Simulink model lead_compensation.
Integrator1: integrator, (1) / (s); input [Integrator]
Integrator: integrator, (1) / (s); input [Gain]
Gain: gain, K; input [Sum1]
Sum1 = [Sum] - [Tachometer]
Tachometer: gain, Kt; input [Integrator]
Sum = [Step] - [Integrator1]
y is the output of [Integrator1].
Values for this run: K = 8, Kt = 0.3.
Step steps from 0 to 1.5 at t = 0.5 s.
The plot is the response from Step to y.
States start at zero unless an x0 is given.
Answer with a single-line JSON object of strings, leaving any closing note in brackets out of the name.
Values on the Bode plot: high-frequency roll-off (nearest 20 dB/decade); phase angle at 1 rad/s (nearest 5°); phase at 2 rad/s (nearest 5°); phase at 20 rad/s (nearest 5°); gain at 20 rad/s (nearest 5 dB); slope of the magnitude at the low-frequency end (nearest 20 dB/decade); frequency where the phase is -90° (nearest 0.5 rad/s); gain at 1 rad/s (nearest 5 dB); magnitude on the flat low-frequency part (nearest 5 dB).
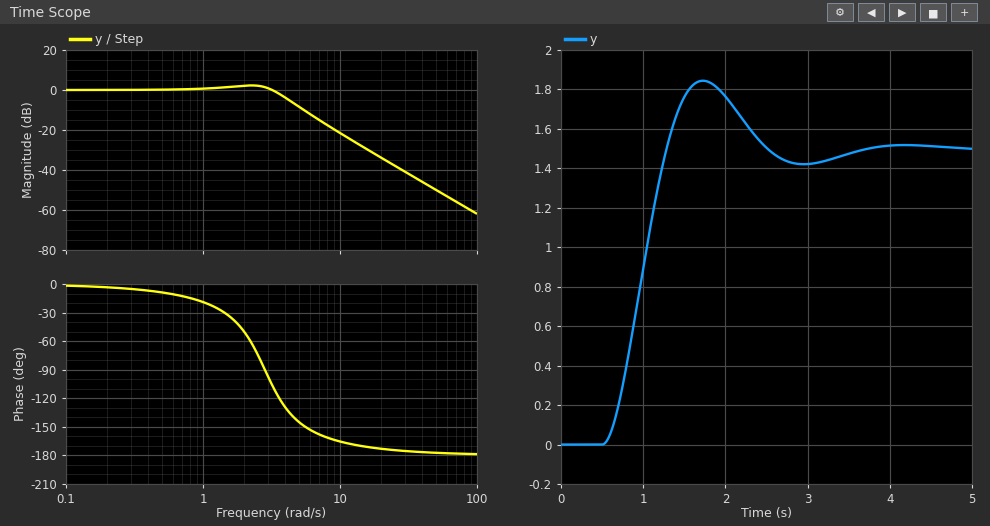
{"high-frequency roll-off": "-40 dB/decade", "phase angle at 1 rad/s": "-20°", "phase at 2 rad/s": "-50°", "phase at 20 rad/s": "-175°", "gain at 20 rad/s": "-35 dB", "slope of the magnitude at the low-frequency end": "0 dB/decade", "frequency where the phase is -90°": "3.0 rad/s", "gain at 1 rad/s": "0 dB", "magnitude on the flat low-frequency part": "0 dB"}
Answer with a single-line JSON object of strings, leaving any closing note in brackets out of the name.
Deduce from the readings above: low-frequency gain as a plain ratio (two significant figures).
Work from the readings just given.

{"low-frequency gain as a plain ratio": "1.0"}
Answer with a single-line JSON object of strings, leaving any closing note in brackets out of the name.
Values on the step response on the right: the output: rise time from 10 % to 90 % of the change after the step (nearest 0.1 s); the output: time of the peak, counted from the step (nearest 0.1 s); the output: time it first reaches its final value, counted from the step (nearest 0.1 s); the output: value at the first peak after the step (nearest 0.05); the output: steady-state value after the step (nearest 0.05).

{"the output: rise time from 10 % to 90 % of the change after the step": "0.5 s", "the output: time of the peak, counted from the step": "1.2 s", "the output: time it first reaches its final value, counted from the step": "0.8 s", "the output: value at the first peak after the step": "1.85", "the output: steady-state value after the step": "1.50"}
